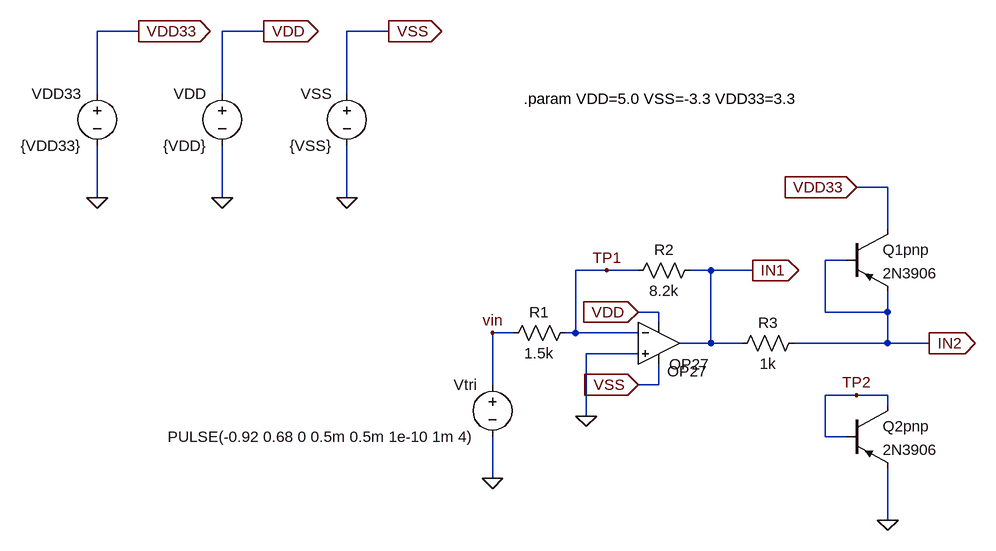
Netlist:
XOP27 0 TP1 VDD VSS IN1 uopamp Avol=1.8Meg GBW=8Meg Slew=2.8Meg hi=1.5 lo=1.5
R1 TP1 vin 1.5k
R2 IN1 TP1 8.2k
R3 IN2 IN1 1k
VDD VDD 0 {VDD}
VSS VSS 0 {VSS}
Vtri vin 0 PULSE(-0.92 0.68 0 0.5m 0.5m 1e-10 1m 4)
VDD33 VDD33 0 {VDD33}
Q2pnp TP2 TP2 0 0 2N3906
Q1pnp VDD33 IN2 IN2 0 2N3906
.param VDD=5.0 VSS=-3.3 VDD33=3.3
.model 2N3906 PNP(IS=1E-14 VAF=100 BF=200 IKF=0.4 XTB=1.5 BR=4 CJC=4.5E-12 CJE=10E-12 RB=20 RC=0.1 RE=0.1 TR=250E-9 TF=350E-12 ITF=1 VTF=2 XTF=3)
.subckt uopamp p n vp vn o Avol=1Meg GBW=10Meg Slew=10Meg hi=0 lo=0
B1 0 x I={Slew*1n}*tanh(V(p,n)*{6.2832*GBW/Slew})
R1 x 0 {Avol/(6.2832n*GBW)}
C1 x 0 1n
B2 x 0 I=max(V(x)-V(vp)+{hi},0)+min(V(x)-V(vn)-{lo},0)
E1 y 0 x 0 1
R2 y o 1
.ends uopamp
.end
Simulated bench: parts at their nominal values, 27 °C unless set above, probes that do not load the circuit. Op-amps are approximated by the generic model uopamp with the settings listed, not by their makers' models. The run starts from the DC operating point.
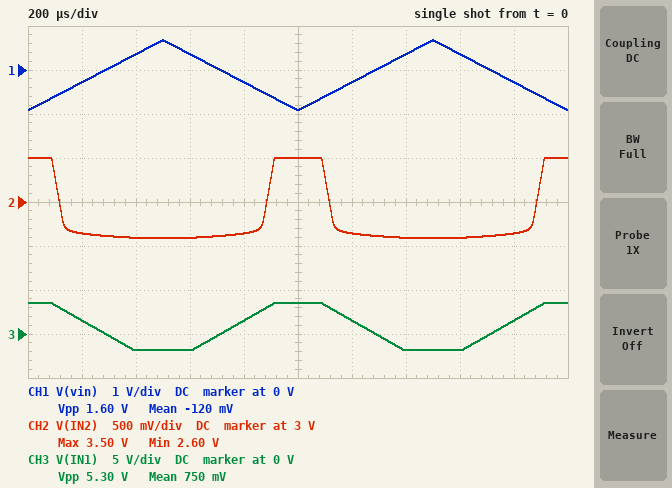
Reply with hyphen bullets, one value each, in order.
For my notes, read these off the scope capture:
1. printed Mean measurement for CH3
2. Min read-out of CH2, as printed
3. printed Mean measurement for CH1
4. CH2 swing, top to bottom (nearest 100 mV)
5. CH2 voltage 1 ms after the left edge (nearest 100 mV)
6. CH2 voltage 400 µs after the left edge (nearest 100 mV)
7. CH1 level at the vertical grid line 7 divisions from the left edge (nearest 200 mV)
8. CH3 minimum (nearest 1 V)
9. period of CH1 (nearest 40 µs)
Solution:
- 750 mV
- 2.60 V
- -120 mV
- 900 mV
- 3.5 V
- 2.6 V
- 400 mV
- -2 V
- 1.00 ms
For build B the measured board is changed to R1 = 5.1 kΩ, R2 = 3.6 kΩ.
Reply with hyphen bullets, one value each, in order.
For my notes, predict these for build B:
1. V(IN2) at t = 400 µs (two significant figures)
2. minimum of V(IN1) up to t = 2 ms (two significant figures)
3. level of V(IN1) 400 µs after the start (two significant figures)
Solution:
- 2.6 V
- -480 mV
- -250 mV
